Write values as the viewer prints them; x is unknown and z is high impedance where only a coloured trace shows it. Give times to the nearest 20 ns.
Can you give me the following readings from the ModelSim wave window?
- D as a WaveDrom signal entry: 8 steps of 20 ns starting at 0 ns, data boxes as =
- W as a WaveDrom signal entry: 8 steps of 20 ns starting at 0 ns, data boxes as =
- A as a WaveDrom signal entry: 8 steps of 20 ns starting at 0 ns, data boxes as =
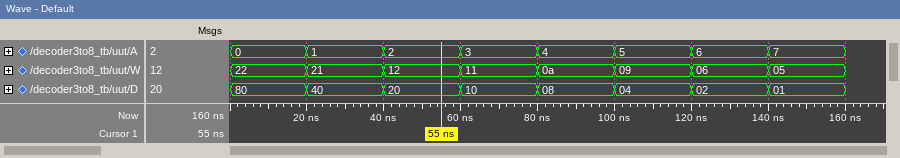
{name: 'D', wave: '========', data: '80 40 20 10 08 04 02 01'}
{name: 'W', wave: '========', data: '22 21 12 11 0a 09 06 05'}
{name: 'A', wave: '========', data: '0 1 2 3 4 5 6 7'}
